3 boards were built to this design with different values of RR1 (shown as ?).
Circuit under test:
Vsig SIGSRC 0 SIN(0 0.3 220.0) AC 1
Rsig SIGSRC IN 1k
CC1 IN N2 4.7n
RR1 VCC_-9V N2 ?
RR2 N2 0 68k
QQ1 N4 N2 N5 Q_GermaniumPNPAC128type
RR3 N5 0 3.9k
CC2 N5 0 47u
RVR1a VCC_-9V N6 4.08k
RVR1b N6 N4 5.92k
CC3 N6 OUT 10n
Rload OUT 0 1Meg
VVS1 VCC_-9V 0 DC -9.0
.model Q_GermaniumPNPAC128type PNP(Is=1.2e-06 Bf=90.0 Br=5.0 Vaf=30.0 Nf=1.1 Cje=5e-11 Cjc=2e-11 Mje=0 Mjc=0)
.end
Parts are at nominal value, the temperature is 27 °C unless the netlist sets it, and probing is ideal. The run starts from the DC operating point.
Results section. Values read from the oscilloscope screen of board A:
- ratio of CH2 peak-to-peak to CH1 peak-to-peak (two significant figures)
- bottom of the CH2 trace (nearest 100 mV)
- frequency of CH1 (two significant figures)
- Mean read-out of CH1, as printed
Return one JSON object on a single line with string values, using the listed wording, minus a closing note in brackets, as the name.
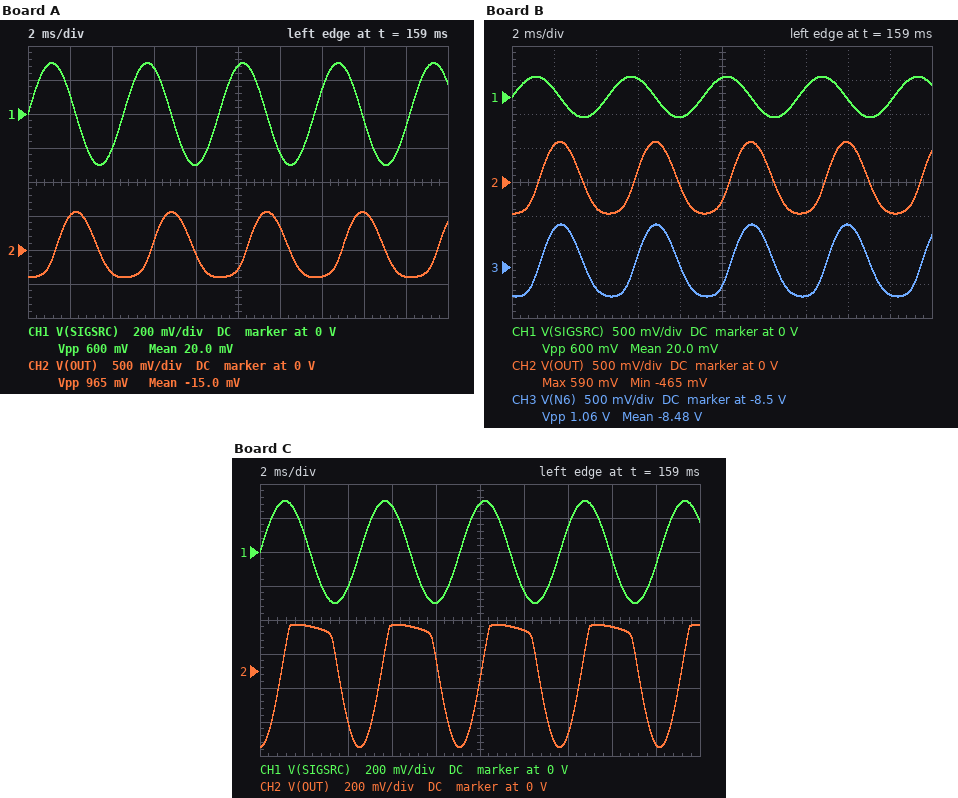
{"ratio of CH2 peak-to-peak to CH1 peak-to-peak": "1.6", "bottom of the CH2 trace": "-400 mV", "frequency of CH1": "220 Hz", "Mean read-out of CH1, as printed": "20.0 mV"}
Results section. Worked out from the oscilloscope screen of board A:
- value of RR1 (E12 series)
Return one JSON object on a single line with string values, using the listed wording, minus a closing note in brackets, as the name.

{"value of RR1": "1 MΩ"}
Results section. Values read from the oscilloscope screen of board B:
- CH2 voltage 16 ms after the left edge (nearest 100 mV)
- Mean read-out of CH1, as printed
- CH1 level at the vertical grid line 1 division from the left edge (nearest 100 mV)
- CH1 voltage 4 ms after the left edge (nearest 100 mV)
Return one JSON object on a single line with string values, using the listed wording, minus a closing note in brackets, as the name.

{"CH2 voltage 16 ms after the left edge": "600 mV", "Mean read-out of CH1, as printed": "20.0 mV", "CH1 level at the vertical grid line 1 division from the left edge": "100 mV", "CH1 voltage 4 ms after the left edge": "-200 mV"}
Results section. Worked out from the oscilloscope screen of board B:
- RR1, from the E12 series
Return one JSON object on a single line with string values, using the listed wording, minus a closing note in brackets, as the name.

{"RR1, from the E12 series": "820 kΩ"}
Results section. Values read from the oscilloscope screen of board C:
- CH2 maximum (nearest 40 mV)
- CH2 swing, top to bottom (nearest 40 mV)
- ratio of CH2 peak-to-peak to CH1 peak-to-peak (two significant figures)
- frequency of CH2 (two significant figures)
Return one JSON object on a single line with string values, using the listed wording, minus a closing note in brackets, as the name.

{"CH2 maximum": "280 mV", "CH2 swing, top to bottom": "720 mV", "ratio of CH2 peak-to-peak to CH1 peak-to-peak": "1.2", "frequency of CH2": "220 Hz"}
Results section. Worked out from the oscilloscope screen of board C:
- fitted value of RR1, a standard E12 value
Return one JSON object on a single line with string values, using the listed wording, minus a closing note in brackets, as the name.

{"fitted value of RR1, a standard E12 value": "150 kΩ"}
